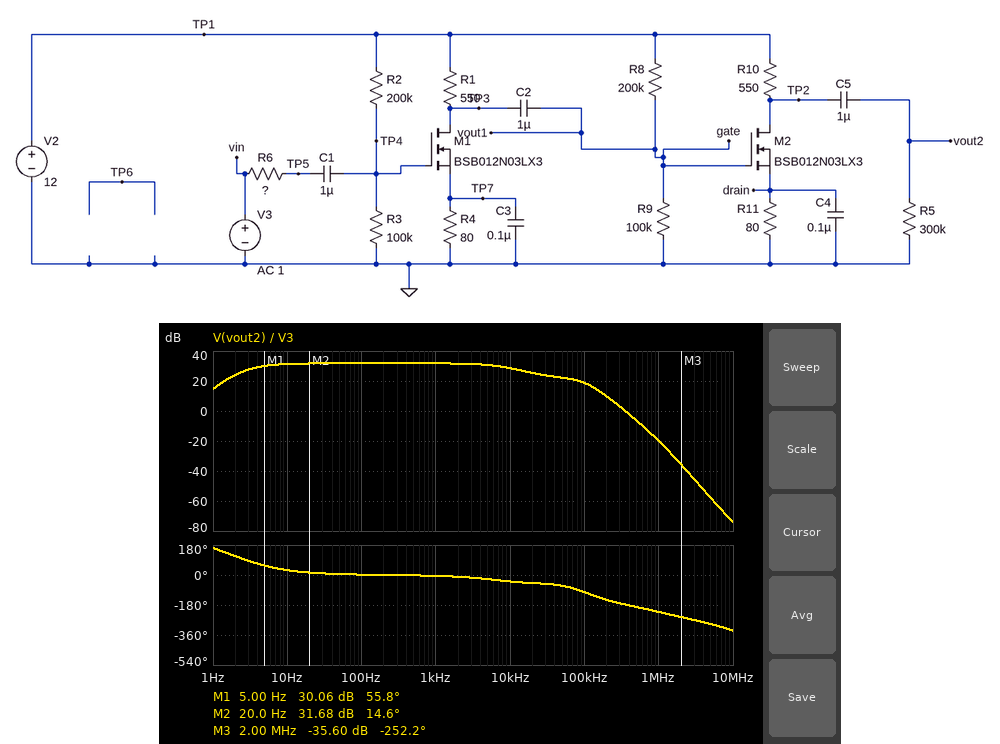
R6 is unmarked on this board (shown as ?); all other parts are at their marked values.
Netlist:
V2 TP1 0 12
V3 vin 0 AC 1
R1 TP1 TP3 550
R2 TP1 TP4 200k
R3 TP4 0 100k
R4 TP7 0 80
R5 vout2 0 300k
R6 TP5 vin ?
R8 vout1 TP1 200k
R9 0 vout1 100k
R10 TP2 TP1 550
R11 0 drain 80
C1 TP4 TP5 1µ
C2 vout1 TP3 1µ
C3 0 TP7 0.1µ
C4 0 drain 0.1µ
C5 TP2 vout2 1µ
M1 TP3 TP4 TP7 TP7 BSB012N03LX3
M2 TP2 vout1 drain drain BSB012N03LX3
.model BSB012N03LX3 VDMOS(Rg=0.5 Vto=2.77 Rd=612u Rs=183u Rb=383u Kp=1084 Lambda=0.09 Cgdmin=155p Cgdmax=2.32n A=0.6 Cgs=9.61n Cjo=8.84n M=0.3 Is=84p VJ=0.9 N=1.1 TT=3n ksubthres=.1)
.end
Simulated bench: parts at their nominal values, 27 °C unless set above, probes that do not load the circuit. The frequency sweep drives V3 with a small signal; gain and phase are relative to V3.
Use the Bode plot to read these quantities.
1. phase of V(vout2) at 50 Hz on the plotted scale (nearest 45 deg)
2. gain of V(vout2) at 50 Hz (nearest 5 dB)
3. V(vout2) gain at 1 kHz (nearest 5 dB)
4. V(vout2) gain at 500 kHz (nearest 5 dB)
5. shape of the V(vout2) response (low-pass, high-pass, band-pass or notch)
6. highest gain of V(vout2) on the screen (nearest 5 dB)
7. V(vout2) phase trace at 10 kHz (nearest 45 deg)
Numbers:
0 deg
30 dB
30 dB
-5 dB
band-pass
30 dB
-45 deg
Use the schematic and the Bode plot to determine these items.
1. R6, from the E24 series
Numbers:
1.1 kΩ
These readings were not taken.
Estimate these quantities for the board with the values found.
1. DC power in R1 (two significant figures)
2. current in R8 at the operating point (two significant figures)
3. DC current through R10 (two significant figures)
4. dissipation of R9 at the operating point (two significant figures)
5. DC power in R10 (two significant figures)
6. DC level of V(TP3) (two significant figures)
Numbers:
200 mW
40 µA
19 mA
160 µW
200 mW
1.6 V
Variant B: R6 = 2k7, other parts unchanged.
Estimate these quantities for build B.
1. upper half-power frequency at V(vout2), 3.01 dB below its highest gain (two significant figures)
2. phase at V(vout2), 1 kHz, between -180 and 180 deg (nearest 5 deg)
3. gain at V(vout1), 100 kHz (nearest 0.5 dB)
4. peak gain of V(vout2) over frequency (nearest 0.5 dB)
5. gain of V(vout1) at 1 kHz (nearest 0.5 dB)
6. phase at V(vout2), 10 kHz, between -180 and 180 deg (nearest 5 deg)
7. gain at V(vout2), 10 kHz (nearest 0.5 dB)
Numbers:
3.6 kHz
-15 deg
-17.0 dB
31.5 dB
15.0 dB
-55 deg
23.0 dB
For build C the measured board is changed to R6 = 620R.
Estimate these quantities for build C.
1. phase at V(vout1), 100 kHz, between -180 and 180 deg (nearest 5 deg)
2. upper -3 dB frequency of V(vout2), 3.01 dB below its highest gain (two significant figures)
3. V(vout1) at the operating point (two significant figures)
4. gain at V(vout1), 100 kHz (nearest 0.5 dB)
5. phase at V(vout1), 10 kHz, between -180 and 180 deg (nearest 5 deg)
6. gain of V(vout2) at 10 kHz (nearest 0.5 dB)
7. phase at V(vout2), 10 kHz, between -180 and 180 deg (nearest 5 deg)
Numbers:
85 deg
19 kHz
4.0 V
-5.0 dB
135 deg
31.0 dB
-25 deg
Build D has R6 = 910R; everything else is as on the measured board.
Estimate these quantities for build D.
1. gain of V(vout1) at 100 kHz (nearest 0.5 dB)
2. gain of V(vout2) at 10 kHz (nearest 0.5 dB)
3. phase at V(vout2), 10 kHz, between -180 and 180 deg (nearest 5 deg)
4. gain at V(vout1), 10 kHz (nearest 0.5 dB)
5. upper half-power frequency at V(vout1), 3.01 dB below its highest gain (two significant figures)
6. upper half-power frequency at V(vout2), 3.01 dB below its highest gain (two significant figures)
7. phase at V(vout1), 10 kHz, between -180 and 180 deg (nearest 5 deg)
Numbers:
-8.0 dB
29.5 dB
-35 deg
12.5 dB
9.4 kHz
12 kHz
125 deg
